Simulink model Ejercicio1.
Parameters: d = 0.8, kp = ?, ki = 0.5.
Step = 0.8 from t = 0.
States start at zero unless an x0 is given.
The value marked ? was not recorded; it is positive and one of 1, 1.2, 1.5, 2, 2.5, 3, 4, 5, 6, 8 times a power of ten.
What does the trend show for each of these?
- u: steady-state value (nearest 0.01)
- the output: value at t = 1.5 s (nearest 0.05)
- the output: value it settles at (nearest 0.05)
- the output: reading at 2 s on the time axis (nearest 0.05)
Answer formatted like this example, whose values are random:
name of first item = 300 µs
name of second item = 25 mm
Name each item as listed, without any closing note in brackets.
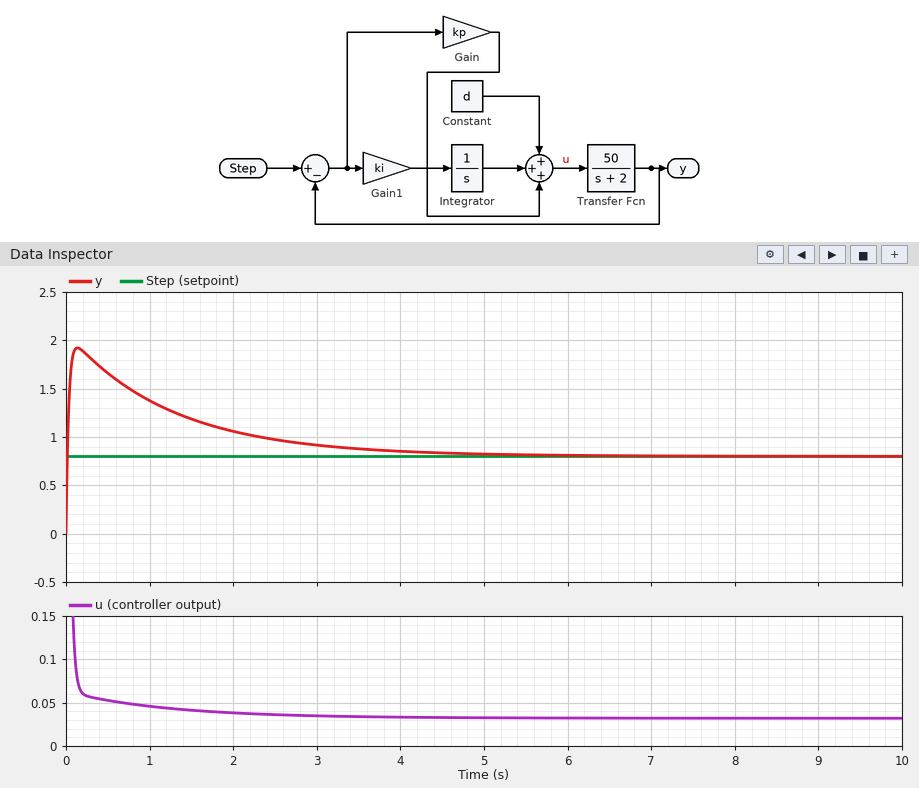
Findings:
u: steady-state value = 0.03
the output: value at t = 1.5 s = 1.20
the output: value it settles at = 0.80
the output: reading at 2 s on the time axis = 1.05
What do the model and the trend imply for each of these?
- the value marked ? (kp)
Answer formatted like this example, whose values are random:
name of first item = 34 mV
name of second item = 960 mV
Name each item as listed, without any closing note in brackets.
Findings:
the value marked ? = 0.6
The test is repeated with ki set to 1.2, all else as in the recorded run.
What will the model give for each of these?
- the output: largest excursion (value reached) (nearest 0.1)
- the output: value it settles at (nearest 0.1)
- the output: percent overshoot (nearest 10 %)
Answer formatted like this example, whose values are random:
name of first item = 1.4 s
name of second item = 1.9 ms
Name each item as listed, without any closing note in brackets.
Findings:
the output: largest excursion (value reached) = 1.9
the output: value it settles at = 0.8
the output: percent overshoot = 130 %
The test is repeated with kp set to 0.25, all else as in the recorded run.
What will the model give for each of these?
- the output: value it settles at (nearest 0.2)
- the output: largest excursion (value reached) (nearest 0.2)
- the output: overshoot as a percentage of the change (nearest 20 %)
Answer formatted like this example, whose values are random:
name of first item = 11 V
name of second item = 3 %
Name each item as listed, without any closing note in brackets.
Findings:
the output: value it settles at = 0.8
the output: largest excursion (value reached) = 3.0
the output: overshoot as a percentage of the change = 280 %
